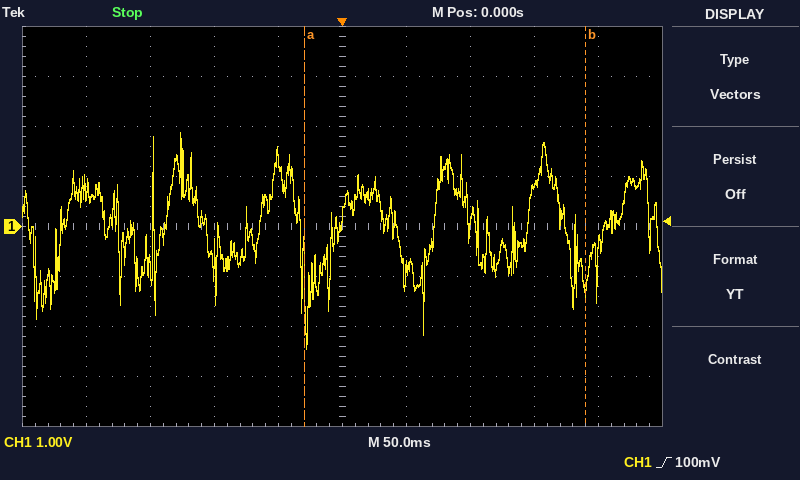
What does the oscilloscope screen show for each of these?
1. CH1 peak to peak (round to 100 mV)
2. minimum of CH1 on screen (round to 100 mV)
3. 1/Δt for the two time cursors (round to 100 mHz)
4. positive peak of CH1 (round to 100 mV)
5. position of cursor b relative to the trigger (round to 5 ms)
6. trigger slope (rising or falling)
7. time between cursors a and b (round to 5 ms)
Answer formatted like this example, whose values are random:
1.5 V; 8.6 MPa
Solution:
4.3 V; -2.4 V; 4.5 Hz; 1.9 V; +190 ms; rising; 220 ms
